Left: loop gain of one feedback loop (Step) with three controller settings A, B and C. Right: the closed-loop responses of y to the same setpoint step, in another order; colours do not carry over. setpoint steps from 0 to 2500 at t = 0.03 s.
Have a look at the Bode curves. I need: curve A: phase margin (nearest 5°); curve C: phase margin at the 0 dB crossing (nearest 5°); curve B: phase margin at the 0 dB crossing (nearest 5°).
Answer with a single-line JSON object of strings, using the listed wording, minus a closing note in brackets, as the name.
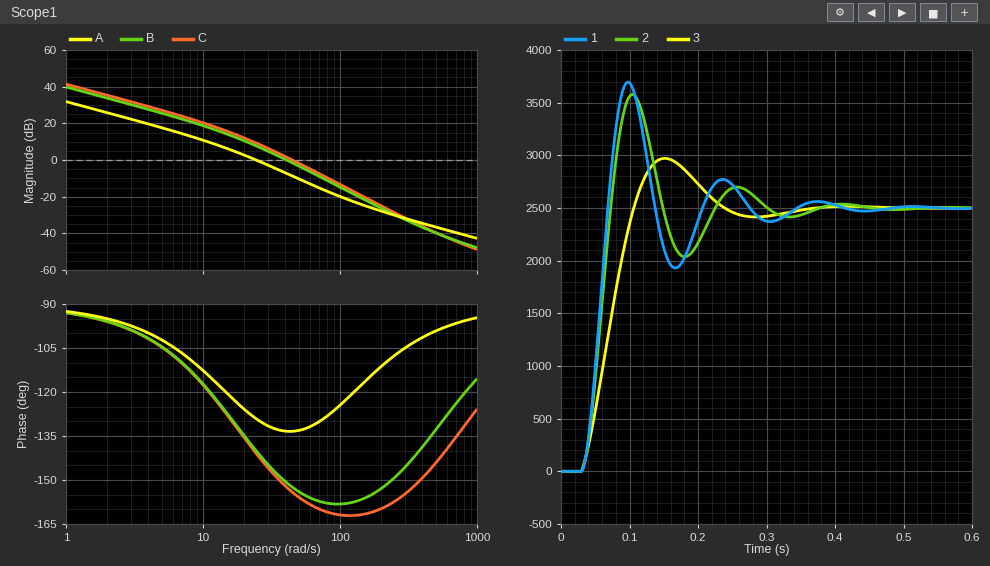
{"curve A: phase margin": "50°", "curve C: phase margin at the 0 dB crossing": "25°", "curve B: phase margin at the 0 dB crossing": "30°"}
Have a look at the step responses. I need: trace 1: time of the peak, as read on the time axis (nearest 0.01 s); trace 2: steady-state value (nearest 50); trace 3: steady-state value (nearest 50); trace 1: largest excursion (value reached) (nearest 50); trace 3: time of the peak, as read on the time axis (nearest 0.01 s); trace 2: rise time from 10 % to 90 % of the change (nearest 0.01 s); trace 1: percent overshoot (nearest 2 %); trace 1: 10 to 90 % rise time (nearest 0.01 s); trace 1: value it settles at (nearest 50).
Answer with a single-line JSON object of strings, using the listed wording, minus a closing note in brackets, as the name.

{"trace 1: time of the peak, as read on the time axis": "0.10 s", "trace 2: steady-state value": "2500", "trace 3: steady-state value": "2500", "trace 1: largest excursion (value reached)": "3700", "trace 3: time of the peak, as read on the time axis": "0.15 s", "trace 2: rise time from 10 % to 90 % of the change": "0.03 s", "trace 1: percent overshoot": "48 %", "trace 1: 10 to 90 % rise time": "0.03 s", "trace 1: value it settles at": "2500"}
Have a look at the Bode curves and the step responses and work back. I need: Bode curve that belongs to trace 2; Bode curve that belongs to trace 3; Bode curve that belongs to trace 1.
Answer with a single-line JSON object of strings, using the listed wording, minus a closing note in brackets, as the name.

{"Bode curve that belongs to trace 2": "B", "Bode curve that belongs to trace 3": "A", "Bode curve that belongs to trace 1": "C"}
